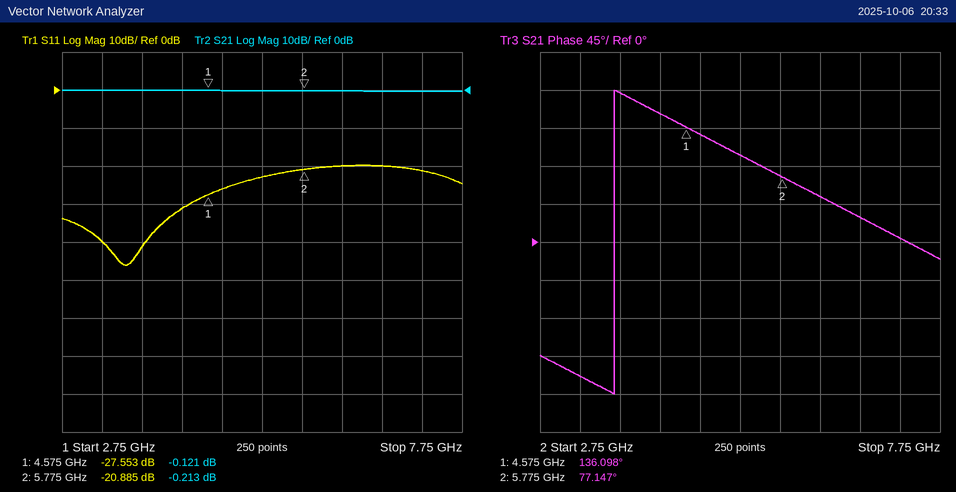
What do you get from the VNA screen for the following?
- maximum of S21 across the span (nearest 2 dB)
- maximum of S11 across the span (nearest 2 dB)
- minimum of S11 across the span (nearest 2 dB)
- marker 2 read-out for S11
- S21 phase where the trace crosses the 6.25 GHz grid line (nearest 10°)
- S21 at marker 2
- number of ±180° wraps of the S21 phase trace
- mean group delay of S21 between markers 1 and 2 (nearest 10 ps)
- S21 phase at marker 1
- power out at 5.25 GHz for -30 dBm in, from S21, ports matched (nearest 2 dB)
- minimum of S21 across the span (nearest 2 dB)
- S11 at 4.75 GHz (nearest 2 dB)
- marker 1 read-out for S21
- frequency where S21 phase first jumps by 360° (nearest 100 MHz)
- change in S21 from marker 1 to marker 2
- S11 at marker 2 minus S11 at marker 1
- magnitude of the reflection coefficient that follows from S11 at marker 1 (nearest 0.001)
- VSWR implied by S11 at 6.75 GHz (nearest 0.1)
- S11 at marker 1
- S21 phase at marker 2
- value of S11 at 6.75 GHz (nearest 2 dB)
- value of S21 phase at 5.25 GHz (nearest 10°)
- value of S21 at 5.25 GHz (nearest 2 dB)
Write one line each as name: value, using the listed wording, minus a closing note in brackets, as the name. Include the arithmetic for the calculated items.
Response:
maximum of S21 across the span: 0 dB
maximum of S11 across the span: -20 dB
minimum of S11 across the span: -46 dB
marker 2 read-out for S11: -20.885 dB
S21 phase where the trace crosses the 6.25 GHz grid line: 50°
S21 at marker 2: -0.213 dB
number of ±180° wraps of the S21 phase trace: 1
mean group delay of S21 between markers 1 and 2: −(77.147° − (136.098°))/(360° × 1.2 GHz) ≈ 136 ps, so 140 ps to the nearest 10 ps
S21 phase at marker 1: 136.098°
power out at 5.25 GHz for -30 dBm in, from S21, ports matched: -30 dBm + (0 dB) = -30 dBm
minimum of S21 across the span: 0 dB
S11 at 4.75 GHz: -26 dB
marker 1 read-out for S21: -0.121 dB
frequency where S21 phase first jumps by 360°: 3.7 GHz
change in S21 from marker 1 to marker 2: -0.213 − (-0.121) = -0.092 dB
S11 at marker 2 minus S11 at marker 1: -20.885 − (-27.553) = 6.668 dB
magnitude of the reflection coefficient that follows from S11 at marker 1: 10^(-27.553/20) ≈ 0.042
VSWR implied by S11 at 6.75 GHz: |Γ| = 10^(-20/20) = 0.1000; VSWR = (1 + 0.1000)/(1 − 0.1000) ≈ 1.2
S11 at marker 1: -27.553 dB
S21 phase at marker 2: 77.147°
value of S11 at 6.75 GHz: -20 dB
value of S21 phase at 5.25 GHz: 100°
value of S21 at 5.25 GHz: 0 dB
